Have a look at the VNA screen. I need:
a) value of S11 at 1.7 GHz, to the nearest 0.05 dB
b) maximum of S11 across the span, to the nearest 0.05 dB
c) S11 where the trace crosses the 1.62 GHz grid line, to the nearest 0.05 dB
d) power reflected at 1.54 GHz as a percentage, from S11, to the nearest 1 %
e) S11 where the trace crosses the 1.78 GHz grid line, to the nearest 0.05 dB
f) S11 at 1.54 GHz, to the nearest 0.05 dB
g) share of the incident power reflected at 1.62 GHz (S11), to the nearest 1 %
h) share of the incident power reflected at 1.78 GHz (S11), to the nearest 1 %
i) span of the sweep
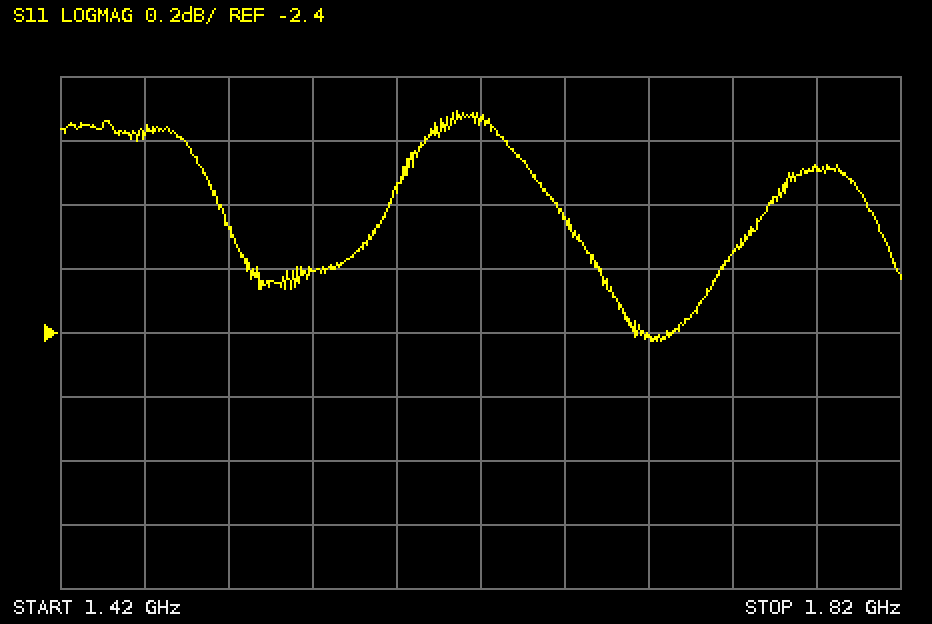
-2.40 dB
-1.70 dB
-1.75 dB
60 %
-1.90 dB
-2.20 dB
67 %
65 %
400 MHz
